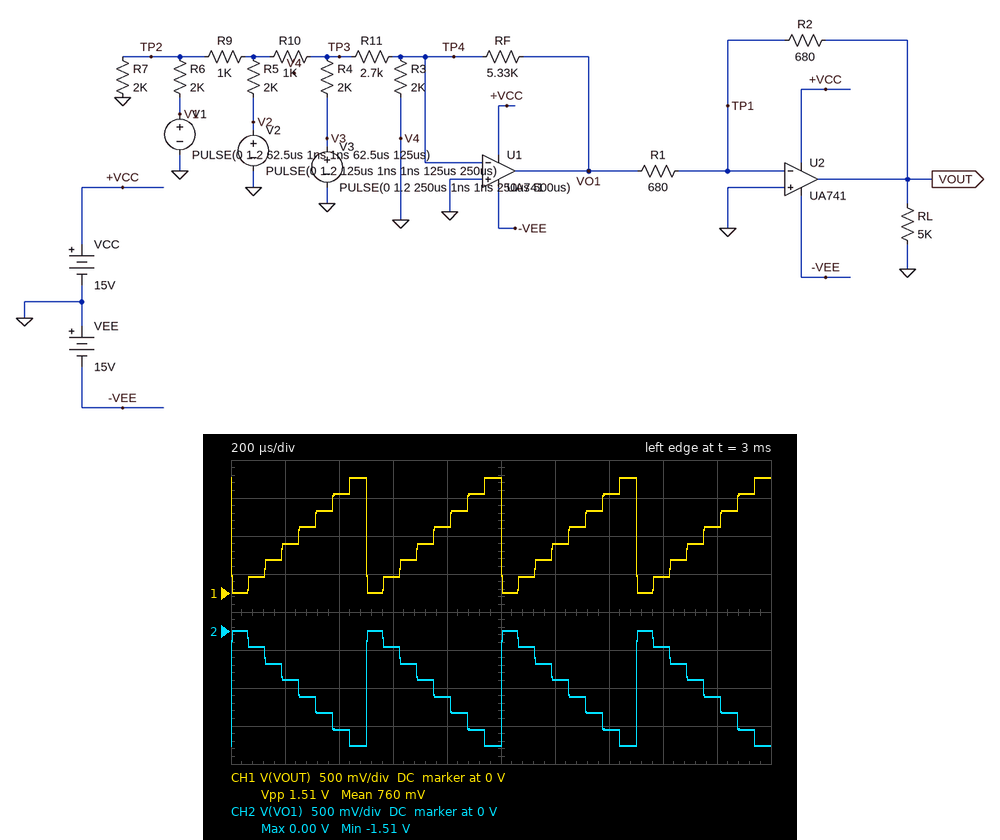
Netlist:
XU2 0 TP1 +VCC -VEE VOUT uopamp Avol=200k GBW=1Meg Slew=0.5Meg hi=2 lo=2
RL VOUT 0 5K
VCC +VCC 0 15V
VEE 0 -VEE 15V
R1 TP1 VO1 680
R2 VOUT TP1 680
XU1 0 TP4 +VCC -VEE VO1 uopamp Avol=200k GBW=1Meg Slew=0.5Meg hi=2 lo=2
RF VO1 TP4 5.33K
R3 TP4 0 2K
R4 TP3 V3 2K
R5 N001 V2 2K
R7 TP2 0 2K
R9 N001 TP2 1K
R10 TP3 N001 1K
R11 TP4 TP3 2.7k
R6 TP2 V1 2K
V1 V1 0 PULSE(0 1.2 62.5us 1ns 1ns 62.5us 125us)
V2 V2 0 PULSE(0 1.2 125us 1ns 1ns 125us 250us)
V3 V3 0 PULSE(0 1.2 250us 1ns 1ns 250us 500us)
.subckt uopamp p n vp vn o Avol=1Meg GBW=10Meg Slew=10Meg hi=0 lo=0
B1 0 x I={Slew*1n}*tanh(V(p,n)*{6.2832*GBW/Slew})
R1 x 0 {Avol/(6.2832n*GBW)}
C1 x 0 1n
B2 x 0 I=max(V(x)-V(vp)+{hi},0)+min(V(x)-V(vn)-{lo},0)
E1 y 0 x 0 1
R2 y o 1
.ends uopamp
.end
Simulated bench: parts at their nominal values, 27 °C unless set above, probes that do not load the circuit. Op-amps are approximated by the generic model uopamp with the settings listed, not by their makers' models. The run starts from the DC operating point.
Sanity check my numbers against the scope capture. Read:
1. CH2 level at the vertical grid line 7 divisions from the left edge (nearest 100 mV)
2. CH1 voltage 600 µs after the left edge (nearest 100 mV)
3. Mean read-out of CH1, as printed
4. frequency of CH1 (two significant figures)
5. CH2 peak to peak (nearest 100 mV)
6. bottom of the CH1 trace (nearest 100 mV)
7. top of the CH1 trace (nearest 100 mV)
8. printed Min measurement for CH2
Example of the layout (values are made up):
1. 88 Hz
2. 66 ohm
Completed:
1. -1.3 V
2. 200 mV
3. 760 mV
4. 2.0 kHz
5. 1.5 V
6. 0 V
7. 1.5 V
8. -1.51 V
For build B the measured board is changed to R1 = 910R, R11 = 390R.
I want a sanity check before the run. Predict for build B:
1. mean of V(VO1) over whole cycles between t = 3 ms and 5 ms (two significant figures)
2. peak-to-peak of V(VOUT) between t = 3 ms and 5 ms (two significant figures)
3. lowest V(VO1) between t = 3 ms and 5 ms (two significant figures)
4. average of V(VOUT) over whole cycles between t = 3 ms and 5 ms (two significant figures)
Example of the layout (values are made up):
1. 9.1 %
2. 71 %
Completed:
1. -2.0 V
2. 3.0 V
3. -4.0 V
4. 1.5 V
